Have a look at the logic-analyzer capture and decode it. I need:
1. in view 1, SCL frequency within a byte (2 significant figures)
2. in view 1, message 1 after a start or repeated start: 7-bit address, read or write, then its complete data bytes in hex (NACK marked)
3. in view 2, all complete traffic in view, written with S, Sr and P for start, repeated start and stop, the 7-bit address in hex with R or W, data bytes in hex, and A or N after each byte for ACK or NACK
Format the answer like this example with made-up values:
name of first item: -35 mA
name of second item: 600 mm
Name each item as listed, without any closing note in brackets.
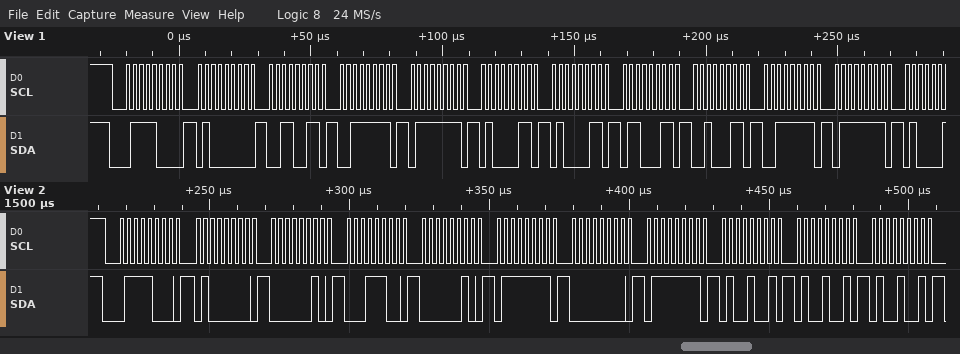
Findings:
in view 1, SCL frequency within a byte: 400 kHz
in view 1, message 1 after a start or repeated start: 7-bit address, read or write, then its complete data bytes in hex: 0x3C write: 40 33 3F 7F 43 43 63 23 3F 7F
in view 2, all complete traffic in view, written with S, Sr and P for start, repeated start and stop, the 7-bit address in hex with R or W, data bytes in hex, and A or N after each byte for ACK or NACK: S 3CW A 40 A 02 A 1C A 02 A 7F A 00 A 7F A 49 A 49 A 49 A
